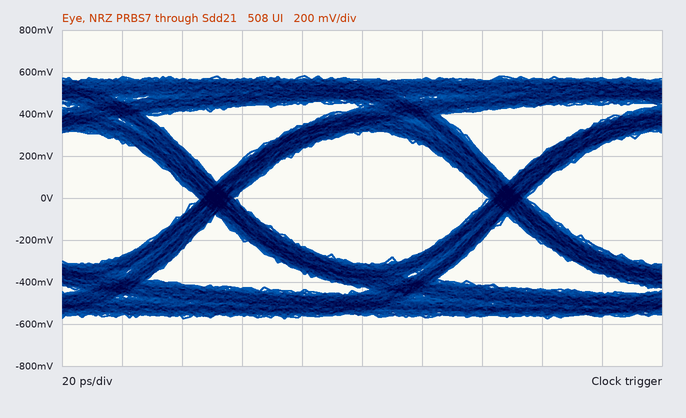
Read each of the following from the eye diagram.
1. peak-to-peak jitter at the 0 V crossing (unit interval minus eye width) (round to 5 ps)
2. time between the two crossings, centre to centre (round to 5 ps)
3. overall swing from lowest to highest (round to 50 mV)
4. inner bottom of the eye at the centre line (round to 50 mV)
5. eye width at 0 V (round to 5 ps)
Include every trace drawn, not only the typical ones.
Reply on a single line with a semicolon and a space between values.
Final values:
10 ps; 95 ps; 1.15 V; -300 mV; 85 ps
